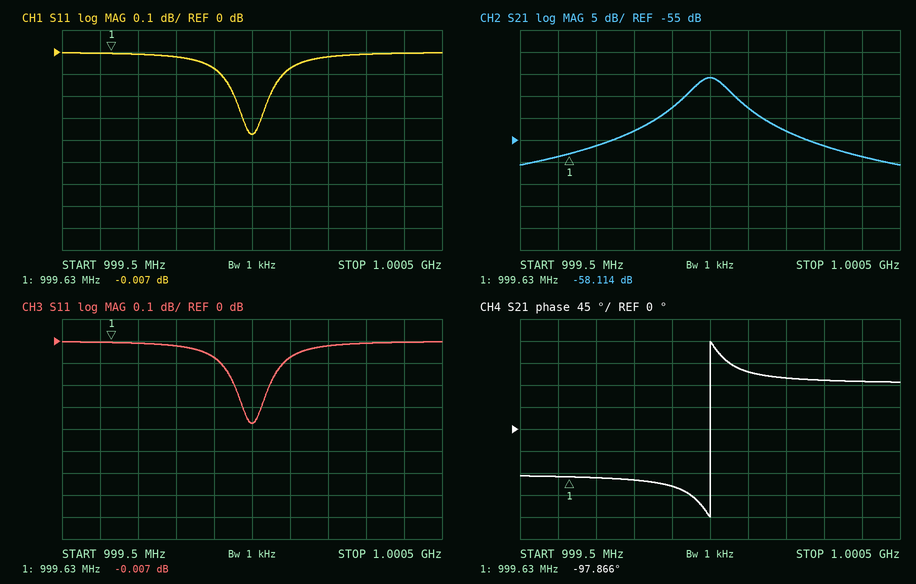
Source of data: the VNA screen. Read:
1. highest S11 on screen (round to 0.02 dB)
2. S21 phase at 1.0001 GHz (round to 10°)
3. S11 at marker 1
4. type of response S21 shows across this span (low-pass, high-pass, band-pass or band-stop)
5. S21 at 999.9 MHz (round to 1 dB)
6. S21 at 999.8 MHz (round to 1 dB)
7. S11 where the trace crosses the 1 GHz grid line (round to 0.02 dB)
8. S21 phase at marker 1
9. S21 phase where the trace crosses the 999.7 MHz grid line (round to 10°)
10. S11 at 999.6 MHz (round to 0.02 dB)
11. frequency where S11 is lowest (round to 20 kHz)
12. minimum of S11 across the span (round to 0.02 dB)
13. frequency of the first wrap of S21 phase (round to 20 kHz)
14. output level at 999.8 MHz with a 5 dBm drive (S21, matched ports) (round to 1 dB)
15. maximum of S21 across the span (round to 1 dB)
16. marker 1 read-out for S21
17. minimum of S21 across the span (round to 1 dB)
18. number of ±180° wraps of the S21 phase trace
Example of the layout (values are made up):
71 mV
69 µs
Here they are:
0.00 dB
120°
-0.007 dB
band-pass
-48 dB
-53 dB
-0.38 dB
-97.866°
-100°
0.00 dB
1.00000 GHz
-0.38 dB
1.00000 GHz
-48 dBm
-41 dB
-58.114 dB
-61 dB
1
